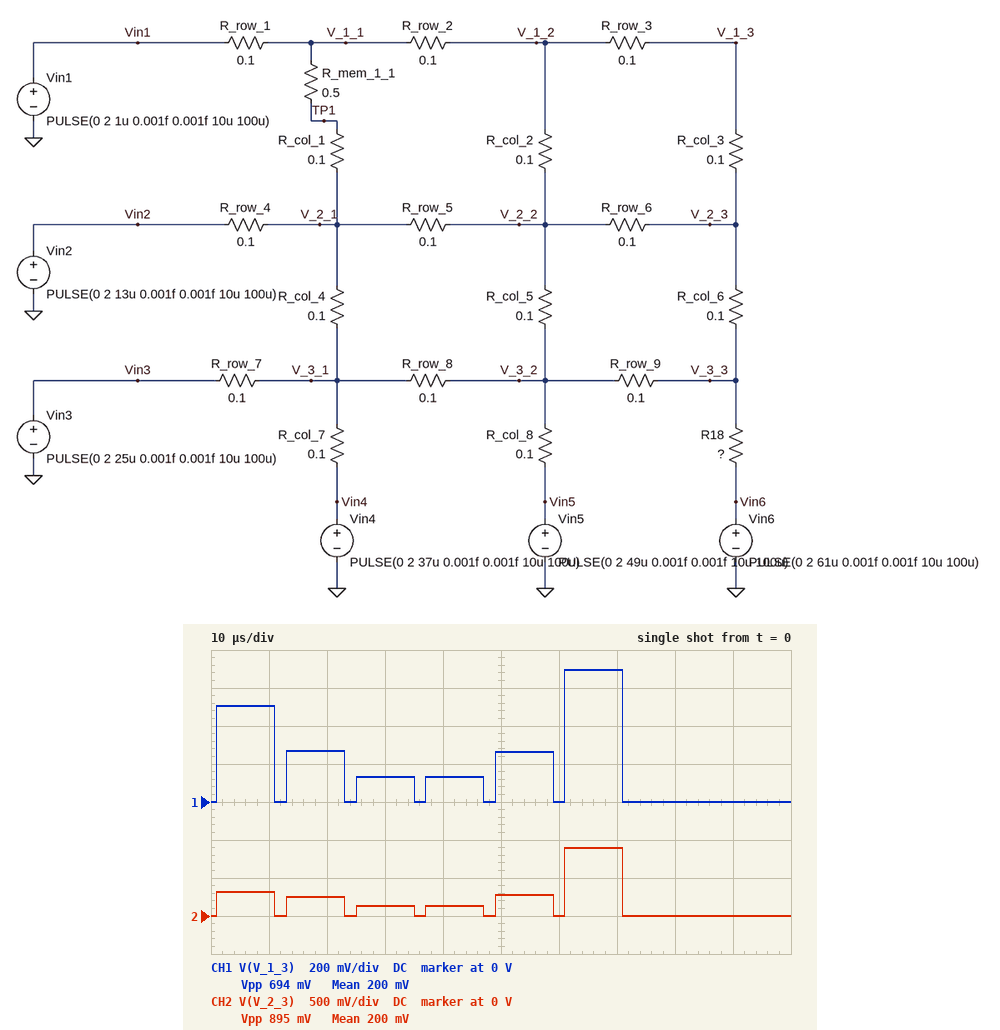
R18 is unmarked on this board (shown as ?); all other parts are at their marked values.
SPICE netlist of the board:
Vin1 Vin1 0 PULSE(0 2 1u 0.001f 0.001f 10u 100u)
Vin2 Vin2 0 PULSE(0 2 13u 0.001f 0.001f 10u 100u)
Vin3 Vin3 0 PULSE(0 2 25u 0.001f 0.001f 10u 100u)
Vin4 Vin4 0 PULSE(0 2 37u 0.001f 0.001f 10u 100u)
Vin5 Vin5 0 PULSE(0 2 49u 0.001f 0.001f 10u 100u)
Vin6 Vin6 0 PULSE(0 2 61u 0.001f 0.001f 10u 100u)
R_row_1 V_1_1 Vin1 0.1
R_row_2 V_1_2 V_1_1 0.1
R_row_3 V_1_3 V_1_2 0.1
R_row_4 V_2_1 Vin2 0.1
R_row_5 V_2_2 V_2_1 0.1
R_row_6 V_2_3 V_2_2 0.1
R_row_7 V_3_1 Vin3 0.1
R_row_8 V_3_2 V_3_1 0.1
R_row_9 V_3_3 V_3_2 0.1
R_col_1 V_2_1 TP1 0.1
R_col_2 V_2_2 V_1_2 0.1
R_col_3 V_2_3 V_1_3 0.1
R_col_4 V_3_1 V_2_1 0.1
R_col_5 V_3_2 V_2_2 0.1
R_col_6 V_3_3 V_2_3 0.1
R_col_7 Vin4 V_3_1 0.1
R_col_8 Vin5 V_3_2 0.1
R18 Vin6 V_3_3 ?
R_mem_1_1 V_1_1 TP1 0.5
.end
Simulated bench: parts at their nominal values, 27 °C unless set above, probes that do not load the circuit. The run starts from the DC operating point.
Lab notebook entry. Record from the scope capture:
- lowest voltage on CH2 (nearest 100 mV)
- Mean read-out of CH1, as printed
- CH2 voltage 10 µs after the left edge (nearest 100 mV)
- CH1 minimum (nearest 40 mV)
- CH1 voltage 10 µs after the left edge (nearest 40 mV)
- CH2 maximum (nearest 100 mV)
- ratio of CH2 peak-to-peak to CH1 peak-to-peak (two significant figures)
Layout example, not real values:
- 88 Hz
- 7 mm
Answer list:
- 0 V
- 200 mV
- 300 mV
- 0 V
- 520 mV
- 900 mV
- 1.3
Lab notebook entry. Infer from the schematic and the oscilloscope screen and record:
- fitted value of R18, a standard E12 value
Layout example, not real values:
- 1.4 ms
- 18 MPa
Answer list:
- 0.039 Ω
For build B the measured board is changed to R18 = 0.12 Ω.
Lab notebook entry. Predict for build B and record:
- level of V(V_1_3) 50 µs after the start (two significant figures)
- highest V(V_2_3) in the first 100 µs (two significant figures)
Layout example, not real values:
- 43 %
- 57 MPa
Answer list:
- 360 mV
- 560 mV
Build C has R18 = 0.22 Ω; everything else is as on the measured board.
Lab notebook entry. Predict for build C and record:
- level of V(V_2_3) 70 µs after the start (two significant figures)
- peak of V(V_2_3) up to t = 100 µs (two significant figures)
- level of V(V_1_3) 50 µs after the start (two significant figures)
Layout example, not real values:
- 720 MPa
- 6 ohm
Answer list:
- 390 mV
- 470 mV
- 410 mV
